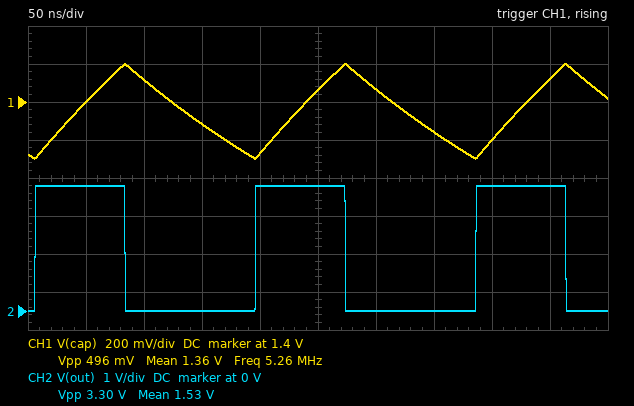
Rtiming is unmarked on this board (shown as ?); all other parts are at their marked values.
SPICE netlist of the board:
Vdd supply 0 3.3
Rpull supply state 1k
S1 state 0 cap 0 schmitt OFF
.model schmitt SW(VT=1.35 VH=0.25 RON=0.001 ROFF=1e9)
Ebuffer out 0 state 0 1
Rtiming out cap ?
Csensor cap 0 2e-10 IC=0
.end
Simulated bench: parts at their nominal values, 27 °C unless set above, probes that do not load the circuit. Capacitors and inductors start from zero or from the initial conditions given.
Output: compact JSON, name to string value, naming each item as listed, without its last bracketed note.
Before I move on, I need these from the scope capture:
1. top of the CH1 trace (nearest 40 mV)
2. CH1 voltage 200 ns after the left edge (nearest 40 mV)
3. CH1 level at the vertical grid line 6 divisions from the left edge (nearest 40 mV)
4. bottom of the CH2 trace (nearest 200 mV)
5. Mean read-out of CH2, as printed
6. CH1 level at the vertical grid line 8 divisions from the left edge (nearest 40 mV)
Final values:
{"top of the CH1 trace": "1.60 V", "CH1 voltage 200 ns after the left edge": "1.12 V", "CH1 level at the vertical grid line 6 divisions from the left edge": "1.48 V", "bottom of the CH2 trace": "0 V", "Mean read-out of CH2, as printed": "1.53 V", "CH1 level at the vertical grid line 8 divisions from the left edge": "1.20 V"}
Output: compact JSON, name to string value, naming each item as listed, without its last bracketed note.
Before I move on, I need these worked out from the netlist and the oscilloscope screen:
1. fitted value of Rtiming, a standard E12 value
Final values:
{"fitted value of Rtiming, a standard E12 value": "1.5 kΩ"}
